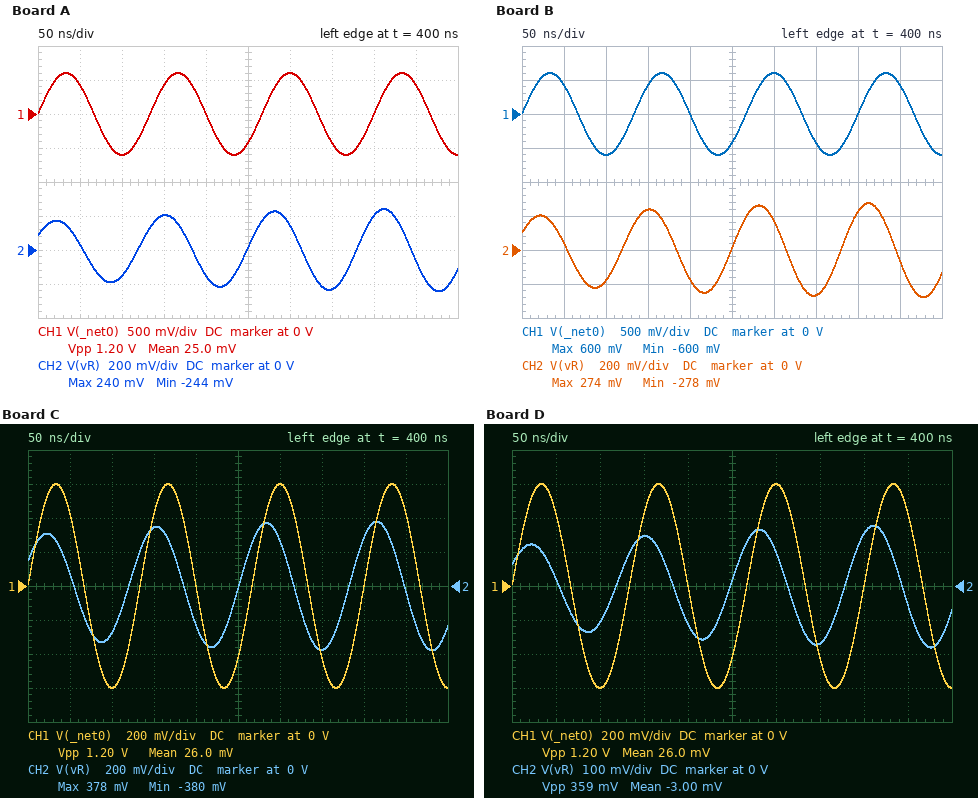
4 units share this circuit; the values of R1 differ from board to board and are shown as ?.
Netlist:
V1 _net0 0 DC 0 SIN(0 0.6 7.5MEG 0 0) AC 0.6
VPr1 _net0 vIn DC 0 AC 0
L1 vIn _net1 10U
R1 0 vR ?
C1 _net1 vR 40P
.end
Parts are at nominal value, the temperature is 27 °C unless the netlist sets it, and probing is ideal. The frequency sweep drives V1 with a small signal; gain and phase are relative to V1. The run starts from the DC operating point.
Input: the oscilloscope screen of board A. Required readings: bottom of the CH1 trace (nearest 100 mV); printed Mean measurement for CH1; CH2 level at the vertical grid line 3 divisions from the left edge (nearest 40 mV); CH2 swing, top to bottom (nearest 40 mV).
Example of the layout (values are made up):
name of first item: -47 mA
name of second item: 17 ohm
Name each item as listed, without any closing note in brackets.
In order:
bottom of the CH1 trace: -600 mV
printed Mean measurement for CH1: 25.0 mV
CH2 level at the vertical grid line 3 divisions from the left edge: 200 mV
CH2 swing, top to bottom: 480 mV
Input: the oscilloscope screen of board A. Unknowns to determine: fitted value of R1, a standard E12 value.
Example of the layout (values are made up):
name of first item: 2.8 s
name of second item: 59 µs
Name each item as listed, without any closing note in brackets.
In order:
fitted value of R1, a standard E12 value: 18 Ω
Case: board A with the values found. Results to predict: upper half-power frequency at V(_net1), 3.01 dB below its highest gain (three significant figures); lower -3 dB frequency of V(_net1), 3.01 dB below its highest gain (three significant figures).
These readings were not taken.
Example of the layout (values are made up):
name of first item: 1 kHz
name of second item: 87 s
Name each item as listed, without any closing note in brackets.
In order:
upper half-power frequency at V(_net1), 3.01 dB below its highest gain: 8.10 MHz
lower -3 dB frequency of V(_net1), 3.01 dB below its highest gain: 7.81 MHz
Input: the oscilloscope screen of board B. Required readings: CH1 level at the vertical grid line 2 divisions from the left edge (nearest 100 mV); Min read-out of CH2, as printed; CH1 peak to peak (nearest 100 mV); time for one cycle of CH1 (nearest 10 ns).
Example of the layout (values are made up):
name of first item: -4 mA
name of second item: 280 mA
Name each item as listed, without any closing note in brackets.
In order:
CH1 level at the vertical grid line 2 divisions from the left edge: -600 mV
Min read-out of CH2, as printed: -278 mV
CH1 peak to peak: 1.2 V
time for one cycle of CH1: 130 ns
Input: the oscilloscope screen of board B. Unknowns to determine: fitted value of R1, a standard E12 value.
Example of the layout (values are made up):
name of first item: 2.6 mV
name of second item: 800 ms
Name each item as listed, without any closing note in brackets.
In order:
fitted value of R1, a standard E12 value: 22 Ω
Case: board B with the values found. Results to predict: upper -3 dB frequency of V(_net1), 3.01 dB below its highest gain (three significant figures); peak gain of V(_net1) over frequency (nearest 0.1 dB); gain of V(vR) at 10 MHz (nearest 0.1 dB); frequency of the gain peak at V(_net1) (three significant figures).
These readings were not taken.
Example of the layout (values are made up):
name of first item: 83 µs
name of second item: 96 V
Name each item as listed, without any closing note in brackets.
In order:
upper -3 dB frequency of V(_net1), 3.01 dB below its highest gain: 8.13 MHz
peak gain of V(_net1) over frequency: 27.1 dB
gain of V(vR) at 10 MHz: -20.4 dB
frequency of the gain peak at V(_net1): 7.95 MHz
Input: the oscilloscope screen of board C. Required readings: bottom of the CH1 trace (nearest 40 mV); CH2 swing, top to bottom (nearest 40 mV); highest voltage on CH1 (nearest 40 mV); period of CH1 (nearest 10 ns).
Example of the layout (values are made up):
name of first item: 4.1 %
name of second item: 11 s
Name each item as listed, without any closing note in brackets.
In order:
bottom of the CH1 trace: -600 mV
CH2 swing, top to bottom: 760 mV
highest voltage on CH1: 600 mV
period of CH1: 130 ns
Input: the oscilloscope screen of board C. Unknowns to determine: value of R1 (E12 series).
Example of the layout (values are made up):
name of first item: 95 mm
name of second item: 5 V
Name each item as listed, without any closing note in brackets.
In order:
value of R1: 39 Ω
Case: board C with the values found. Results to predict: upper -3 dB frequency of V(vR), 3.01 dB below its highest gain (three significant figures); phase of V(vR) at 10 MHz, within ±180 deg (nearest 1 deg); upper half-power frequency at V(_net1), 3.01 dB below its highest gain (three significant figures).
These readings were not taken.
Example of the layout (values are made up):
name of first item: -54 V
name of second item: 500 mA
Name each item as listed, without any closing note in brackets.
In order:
upper -3 dB frequency of V(vR), 3.01 dB below its highest gain: 8.27 MHz
phase of V(vR) at 10 MHz, within ±180 deg: -80 deg
upper half-power frequency at V(_net1), 3.01 dB below its highest gain: 8.25 MHz
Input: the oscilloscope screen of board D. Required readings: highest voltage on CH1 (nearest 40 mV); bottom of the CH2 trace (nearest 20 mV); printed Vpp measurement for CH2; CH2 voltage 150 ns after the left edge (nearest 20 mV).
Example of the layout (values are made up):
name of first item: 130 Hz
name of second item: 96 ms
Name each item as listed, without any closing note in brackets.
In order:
highest voltage on CH1: 600 mV
bottom of the CH2 trace: -180 mV
printed Vpp measurement for CH2: 359 mV
CH2 voltage 150 ns after the left edge: 140 mV
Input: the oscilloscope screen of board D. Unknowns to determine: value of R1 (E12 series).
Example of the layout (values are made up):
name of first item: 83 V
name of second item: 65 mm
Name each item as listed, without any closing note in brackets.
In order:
value of R1: 12 Ω
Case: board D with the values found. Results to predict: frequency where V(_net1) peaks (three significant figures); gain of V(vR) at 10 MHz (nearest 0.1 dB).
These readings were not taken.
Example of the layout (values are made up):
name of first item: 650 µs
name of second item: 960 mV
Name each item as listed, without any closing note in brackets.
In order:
frequency where V(_net1) peaks: 7.96 MHz
gain of V(vR) at 10 MHz: -25.7 dB
